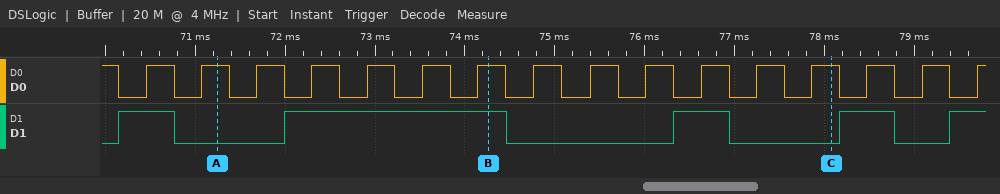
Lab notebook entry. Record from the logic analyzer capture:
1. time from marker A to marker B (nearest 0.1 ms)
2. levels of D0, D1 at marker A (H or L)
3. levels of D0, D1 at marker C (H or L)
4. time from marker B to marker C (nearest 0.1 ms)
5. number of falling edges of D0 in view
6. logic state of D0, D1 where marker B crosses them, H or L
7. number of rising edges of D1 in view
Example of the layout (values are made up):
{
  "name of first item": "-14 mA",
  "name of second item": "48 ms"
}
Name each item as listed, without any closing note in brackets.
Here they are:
{
  "time from marker A to marker B": "3 ms",
  "levels of D0, D1 at marker A": "D0=H, D1=L",
  "levels of D0, D1 at marker C": "D0=H, D1=L",
  "time from marker B to marker C": "3.8 ms",
  "number of falling edges of D0 in view": "16",
  "logic state of D0, D1 where marker B crosses them, H or L": "D0=H, D1=H",
  "number of rising edges of D1 in view": "5"
}
